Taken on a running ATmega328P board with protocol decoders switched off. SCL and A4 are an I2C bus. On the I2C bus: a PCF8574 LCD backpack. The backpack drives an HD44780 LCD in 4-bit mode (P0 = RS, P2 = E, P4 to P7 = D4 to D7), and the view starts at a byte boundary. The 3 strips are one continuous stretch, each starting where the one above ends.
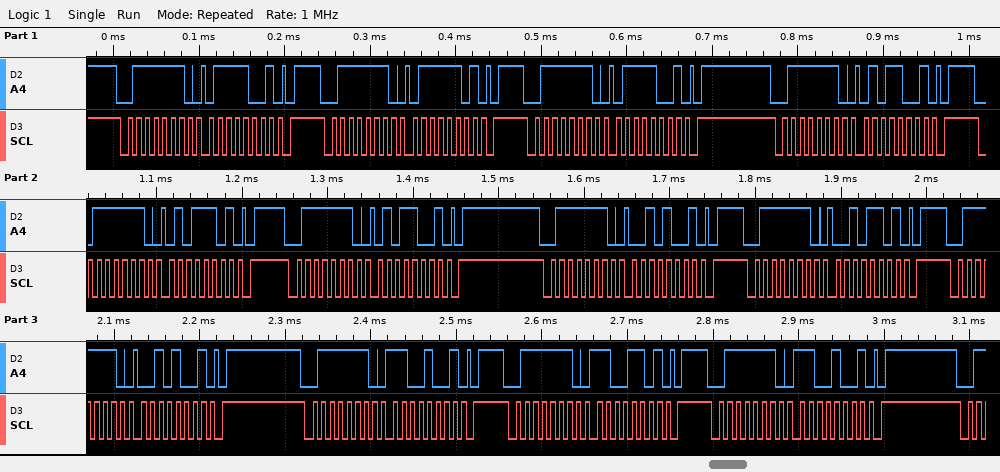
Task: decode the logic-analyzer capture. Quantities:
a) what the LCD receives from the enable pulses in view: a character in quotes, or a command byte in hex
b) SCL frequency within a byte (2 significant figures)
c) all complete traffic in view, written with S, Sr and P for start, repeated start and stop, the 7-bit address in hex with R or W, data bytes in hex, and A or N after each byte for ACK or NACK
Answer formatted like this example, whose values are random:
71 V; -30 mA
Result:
'u' ','; 100 kHz; S 3FW A 79 A P S 3FW A 7D A P S 3FW A 79 A P S 3FW A 59 A P S 3FW A 5D A P S 3FW A 59 A P S 3FW A 29 A P S 3FW A 2D A P S 3FW A 29 A P S 3FW A C9 A P S 3FW A CD A P S 3FW A C9 A P
